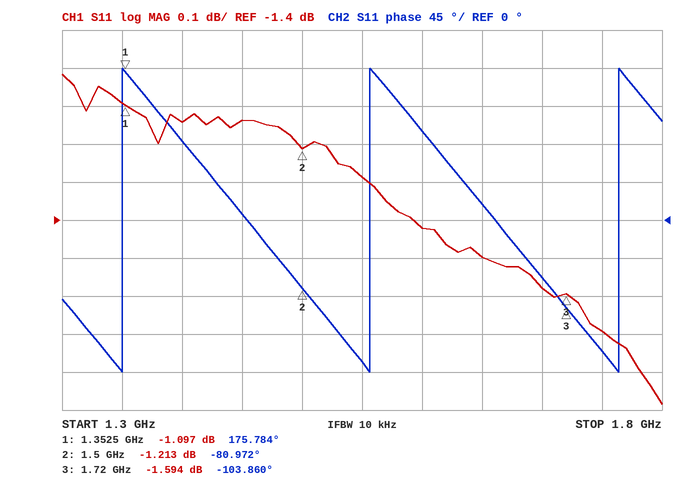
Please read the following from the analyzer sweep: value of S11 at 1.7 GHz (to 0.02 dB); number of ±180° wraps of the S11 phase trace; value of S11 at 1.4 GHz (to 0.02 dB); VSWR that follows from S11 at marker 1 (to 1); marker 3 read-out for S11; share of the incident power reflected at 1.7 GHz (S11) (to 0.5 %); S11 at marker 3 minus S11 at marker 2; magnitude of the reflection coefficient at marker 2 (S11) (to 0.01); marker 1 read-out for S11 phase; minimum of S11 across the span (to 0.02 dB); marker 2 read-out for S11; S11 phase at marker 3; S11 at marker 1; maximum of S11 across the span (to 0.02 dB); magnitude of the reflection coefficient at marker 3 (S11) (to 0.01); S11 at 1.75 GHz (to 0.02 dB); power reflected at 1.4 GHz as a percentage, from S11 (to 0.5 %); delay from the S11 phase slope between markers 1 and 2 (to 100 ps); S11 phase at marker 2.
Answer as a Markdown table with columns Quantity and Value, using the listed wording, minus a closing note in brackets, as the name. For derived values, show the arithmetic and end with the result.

| Quantity | Value |
|---|---|
| value of S11 at 1.7 GHz | -1.58 dB |
| number of ±180° wraps of the S11 phase trace | 3 |
| value of S11 at 1.4 GHz | -1.14 dB |
| VSWR that follows from S11 at marker 1 | (1 + 0.8814)/(1 − 0.8814) ≈ 16 |
| marker 3 read-out for S11 | -1.594 dB |
| share of the incident power reflected at 1.7 GHz (S11) | 10^(-1.58/10) ≈ 69.5 % |
| S11 at marker 3 minus S11 at marker 2 | -1.594 − (-1.213) = -0.381 dB |
| magnitude of the reflection coefficient at marker 2 (S11) | 10^(-1.213/20) ≈ 0.87 |
| marker 1 read-out for S11 phase | 175.784° |
| minimum of S11 across the span | -1.88 dB |
| marker 2 read-out for S11 | -1.213 dB |
| S11 phase at marker 3 | -103.860° |
| S11 at marker 1 | -1.097 dB |
| maximum of S11 across the span | -1.02 dB |
| magnitude of the reflection coefficient at marker 3 (S11) | 10^(-1.594/20) ≈ 0.83 |
| S11 at 1.75 GHz | -1.70 dB |
| power reflected at 1.4 GHz as a percentage, from S11 | 10^(-1.14/10) ≈ 76.9 %, so 77.0 % to the nearest 0.5 % |
| delay from the S11 phase slope between markers 1 and 2 | −(-80.972° − (175.784°))/(360° × 147.5 MHz) ≈ 4.8 ns |
| S11 phase at marker 2 | -80.972° |
